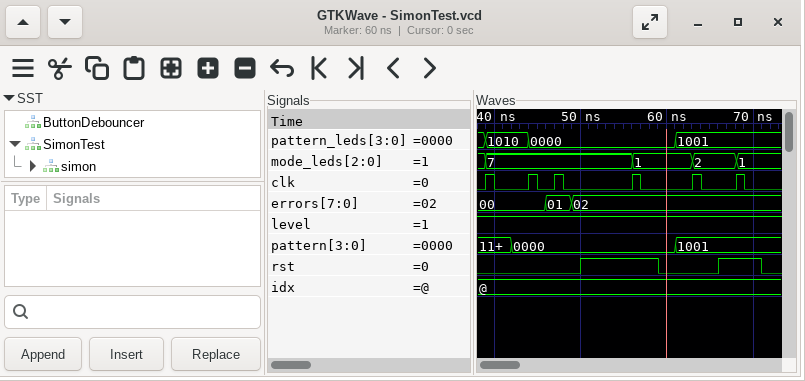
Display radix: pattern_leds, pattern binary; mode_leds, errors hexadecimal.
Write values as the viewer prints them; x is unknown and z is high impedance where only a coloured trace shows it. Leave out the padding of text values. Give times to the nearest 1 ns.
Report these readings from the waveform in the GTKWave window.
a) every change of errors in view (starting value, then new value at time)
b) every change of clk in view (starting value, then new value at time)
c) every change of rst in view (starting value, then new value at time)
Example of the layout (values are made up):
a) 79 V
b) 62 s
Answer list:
a) 00, 01 at 46 ns, 02 at 49 ns
b) 0, 1 at 39 ns, 0 at 40 ns, 1 at 44 ns, 0 at 45 ns, 1 at 47 ns, 0 at 48 ns, 1 at 56 ns, 0 at 57 ns, 1 at 63 ns, 0 at 64 ns, 1 at 68 ns, 0 at 69 ns
c) 0, 1 at 50 ns, 0 at 59 ns, 1 at 66 ns, 0 at 71 ns
